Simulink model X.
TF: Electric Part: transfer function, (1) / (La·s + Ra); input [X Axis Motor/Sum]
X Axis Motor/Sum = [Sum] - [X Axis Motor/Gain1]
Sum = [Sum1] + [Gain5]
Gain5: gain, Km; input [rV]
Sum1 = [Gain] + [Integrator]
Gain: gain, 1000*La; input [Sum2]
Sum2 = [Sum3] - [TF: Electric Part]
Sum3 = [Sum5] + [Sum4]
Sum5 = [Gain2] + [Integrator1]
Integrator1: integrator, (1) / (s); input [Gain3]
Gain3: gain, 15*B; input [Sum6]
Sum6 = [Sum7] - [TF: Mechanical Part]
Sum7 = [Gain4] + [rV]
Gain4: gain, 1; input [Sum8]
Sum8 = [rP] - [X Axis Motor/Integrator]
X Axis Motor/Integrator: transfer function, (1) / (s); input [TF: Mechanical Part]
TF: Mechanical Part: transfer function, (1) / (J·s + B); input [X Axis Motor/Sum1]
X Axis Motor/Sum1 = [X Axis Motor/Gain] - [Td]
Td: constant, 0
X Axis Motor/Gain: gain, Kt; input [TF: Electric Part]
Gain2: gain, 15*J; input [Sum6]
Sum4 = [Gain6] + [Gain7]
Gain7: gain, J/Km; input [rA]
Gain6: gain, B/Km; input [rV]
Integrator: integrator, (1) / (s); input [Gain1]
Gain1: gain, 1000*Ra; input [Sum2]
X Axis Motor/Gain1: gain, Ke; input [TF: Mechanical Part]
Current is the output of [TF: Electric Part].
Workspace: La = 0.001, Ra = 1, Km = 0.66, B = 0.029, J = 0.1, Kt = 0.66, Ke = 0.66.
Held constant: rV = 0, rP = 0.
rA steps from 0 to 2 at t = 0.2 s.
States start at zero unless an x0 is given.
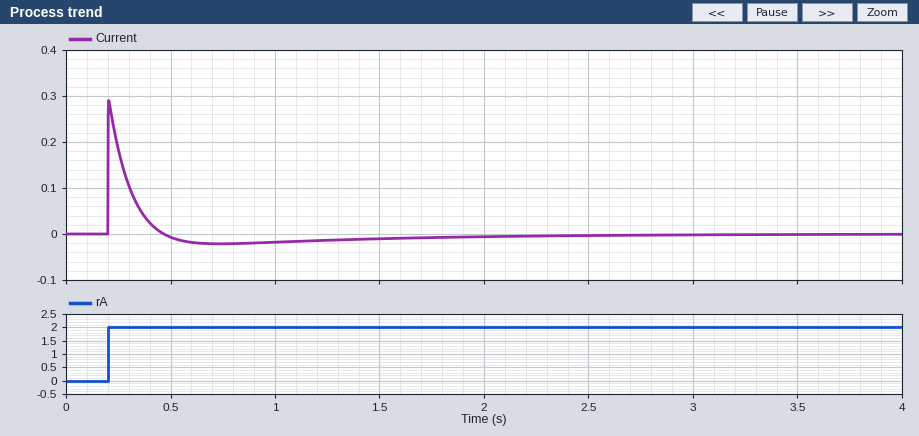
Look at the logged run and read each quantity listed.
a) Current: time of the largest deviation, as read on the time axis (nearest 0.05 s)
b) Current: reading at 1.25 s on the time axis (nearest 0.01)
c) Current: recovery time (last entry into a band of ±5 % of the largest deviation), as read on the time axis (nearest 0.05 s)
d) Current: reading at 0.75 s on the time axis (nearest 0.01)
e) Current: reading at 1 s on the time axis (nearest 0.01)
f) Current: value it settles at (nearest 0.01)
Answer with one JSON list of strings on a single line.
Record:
["0.20 s", "-0.01", "1.20 s", "-0.02", "-0.02", "0.00"]
